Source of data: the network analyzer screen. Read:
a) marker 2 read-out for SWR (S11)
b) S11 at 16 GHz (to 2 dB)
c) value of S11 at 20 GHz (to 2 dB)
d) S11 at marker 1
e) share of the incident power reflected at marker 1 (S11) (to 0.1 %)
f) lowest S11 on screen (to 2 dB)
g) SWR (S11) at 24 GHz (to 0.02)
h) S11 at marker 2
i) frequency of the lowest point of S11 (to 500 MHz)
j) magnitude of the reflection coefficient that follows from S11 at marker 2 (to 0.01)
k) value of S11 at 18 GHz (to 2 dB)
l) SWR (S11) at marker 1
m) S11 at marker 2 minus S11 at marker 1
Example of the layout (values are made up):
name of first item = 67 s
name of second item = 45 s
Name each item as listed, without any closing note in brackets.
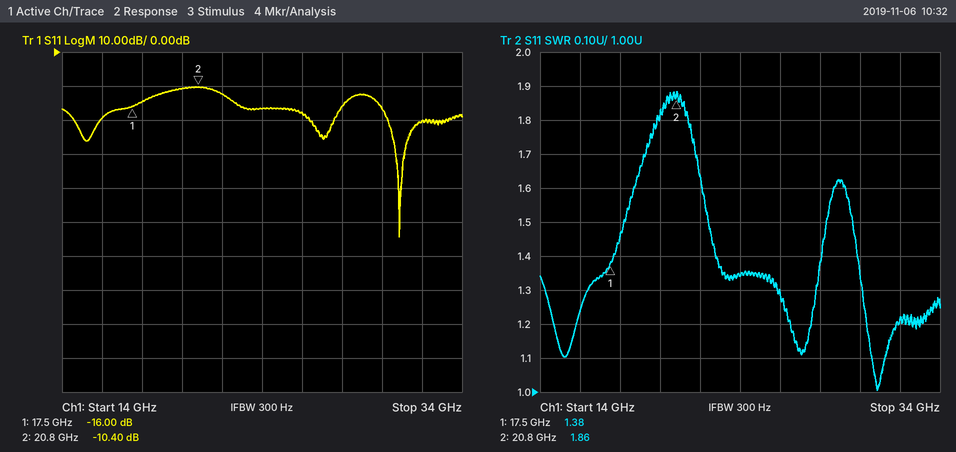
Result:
marker 2 read-out for SWR = 1.86
S11 at 16 GHz = -20 dB
value of S11 at 20 GHz = -10 dB
S11 at marker 1 = -16.00 dB
share of the incident power reflected at marker 1 (S11) = 2.5 %
lowest S11 on screen = -54 dB
SWR (S11) at 24 GHz = 1.34
S11 at marker 2 = -10.40 dB
frequency of the lowest point of S11 = 31.0 GHz
magnitude of the reflection coefficient that follows from S11 at marker 2 = 0.30
value of S11 at 18 GHz = -14 dB
SWR (S11) at marker 1 = 1.38
S11 at marker 2 minus S11 at marker 1 = 5.60 dB
